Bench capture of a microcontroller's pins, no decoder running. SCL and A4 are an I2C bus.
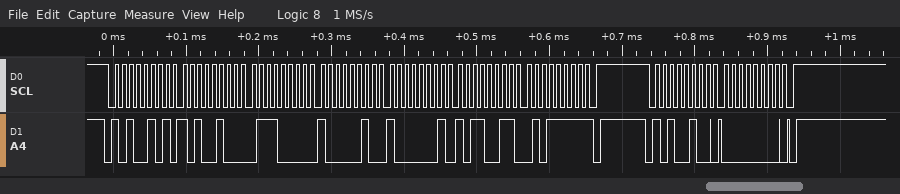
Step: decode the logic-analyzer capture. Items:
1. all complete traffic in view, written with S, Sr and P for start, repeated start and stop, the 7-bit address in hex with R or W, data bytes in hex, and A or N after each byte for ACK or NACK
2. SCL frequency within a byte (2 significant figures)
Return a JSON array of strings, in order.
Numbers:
["S 52R A A4 A 70 A 82 A 81 A B3 A 5F N P S 52W A 00 A P", "100 kHz"]
